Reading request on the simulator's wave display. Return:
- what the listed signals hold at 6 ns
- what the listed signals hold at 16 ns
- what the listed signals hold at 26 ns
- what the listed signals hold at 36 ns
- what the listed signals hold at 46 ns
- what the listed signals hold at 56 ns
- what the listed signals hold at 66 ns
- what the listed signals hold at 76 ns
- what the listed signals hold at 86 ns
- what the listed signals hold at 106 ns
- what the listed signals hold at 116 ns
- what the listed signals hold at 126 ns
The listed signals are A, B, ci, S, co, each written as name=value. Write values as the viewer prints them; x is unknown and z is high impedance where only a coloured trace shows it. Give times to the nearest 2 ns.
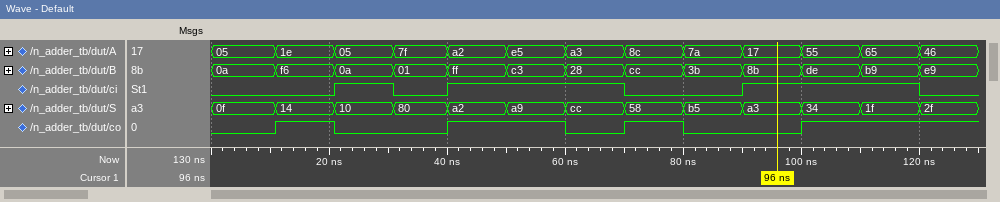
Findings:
A=05, B=0a, ci=0, S=0f, co=0
A=1e, B=f6, ci=0, S=14, co=1
A=05, B=0a, ci=1, S=10, co=0
A=7f, B=01, ci=0, S=80, co=0
A=a2, B=ff, ci=1, S=a2, co=1
A=e5, B=c3, ci=1, S=a9, co=1
A=a3, B=28, ci=1, S=cc, co=0
A=8c, B=cc, ci=0, S=58, co=1
A=7a, B=3b, ci=0, S=b5, co=0
A=55, B=de, ci=1, S=34, co=1
A=65, B=b9, ci=1, S=1f, co=1
A=46, B=e9, ci=0, S=2f, co=1
